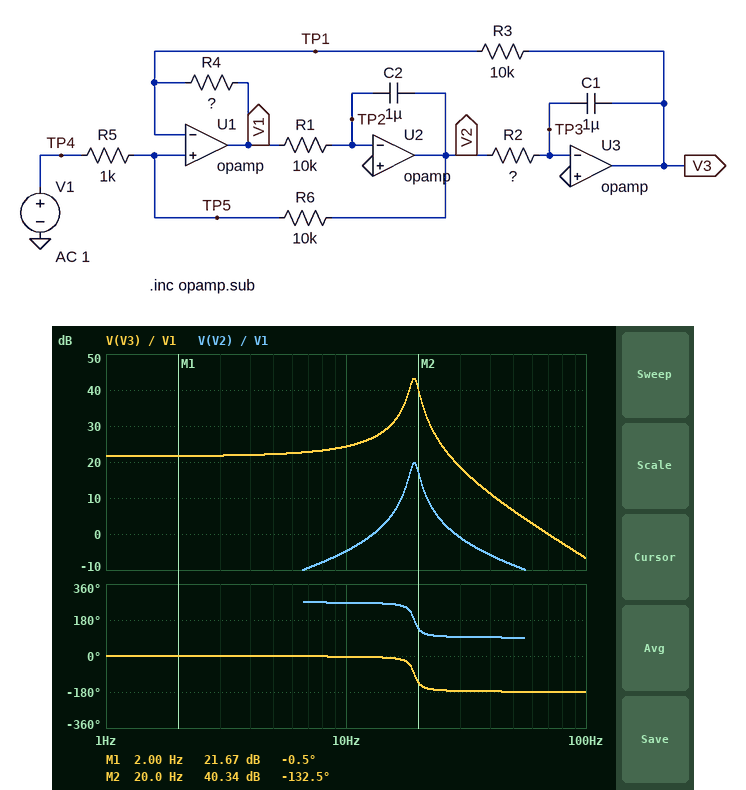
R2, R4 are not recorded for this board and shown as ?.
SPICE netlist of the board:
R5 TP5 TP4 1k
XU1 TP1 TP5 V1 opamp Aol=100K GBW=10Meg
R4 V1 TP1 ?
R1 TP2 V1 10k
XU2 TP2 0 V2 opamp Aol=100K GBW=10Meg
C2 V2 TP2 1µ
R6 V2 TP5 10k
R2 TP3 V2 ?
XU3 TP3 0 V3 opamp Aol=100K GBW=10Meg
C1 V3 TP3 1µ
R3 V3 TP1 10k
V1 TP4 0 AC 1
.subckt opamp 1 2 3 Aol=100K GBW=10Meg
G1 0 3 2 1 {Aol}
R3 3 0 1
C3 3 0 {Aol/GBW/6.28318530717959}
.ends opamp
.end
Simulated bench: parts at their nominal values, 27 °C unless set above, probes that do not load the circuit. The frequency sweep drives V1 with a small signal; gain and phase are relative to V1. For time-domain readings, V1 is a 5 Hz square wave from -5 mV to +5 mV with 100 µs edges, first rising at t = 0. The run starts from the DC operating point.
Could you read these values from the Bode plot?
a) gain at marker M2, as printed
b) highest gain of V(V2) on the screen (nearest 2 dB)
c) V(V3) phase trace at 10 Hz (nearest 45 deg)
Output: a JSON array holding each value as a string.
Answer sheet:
["40.34 dB", "20 dB", "0 deg"]
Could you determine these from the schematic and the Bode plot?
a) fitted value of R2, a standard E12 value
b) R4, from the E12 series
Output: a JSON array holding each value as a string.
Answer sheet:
["560 Ω", "820 Ω"]
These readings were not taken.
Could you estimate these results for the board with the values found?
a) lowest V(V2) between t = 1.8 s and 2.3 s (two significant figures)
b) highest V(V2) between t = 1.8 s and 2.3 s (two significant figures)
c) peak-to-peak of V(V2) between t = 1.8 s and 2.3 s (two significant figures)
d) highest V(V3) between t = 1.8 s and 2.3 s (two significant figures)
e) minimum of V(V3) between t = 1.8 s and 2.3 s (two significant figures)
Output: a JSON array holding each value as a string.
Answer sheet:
["-4.9 mV", "4.9 mV", "9.8 mV", "130 mV", "-130 mV"]
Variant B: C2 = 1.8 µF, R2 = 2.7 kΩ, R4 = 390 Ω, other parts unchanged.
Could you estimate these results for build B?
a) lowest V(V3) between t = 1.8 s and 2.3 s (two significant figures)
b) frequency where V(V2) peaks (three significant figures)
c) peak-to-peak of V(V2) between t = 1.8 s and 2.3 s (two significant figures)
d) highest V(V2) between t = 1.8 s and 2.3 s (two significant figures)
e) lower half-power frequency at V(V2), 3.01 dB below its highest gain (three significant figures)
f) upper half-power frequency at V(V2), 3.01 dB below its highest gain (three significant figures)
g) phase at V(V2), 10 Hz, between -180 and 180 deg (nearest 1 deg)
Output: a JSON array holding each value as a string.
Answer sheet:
["-500 mV", "4.51 Hz", "83 mV", "41 mV", "4.11 Hz", "4.95 Hz", "96 deg"]
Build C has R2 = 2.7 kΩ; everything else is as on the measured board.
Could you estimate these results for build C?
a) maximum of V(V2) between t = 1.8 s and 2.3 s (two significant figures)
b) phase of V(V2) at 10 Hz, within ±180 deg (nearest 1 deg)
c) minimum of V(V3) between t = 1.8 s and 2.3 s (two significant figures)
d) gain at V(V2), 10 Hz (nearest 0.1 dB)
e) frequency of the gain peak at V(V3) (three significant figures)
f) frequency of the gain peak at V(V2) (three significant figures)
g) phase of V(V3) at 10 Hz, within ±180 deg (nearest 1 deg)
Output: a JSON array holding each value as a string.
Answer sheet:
["11 mV", "124 deg", "-120 mV", "15.0 dB", "8.70 Hz", "8.77 Hz", "-146 deg"]
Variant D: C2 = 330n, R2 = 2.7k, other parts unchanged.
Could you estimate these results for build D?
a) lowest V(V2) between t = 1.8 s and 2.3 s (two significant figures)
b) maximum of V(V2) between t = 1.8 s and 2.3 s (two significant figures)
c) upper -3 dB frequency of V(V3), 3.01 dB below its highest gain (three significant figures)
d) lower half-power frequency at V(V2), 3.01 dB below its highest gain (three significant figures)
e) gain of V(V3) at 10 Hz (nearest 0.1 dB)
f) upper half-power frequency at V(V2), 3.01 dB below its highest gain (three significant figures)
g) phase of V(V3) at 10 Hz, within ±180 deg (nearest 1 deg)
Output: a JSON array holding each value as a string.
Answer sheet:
["-32 mV", "32 mV", "17.1 Hz", "13.1 Hz", "25.9 dB", "17.8 Hz", "-20 deg"]
